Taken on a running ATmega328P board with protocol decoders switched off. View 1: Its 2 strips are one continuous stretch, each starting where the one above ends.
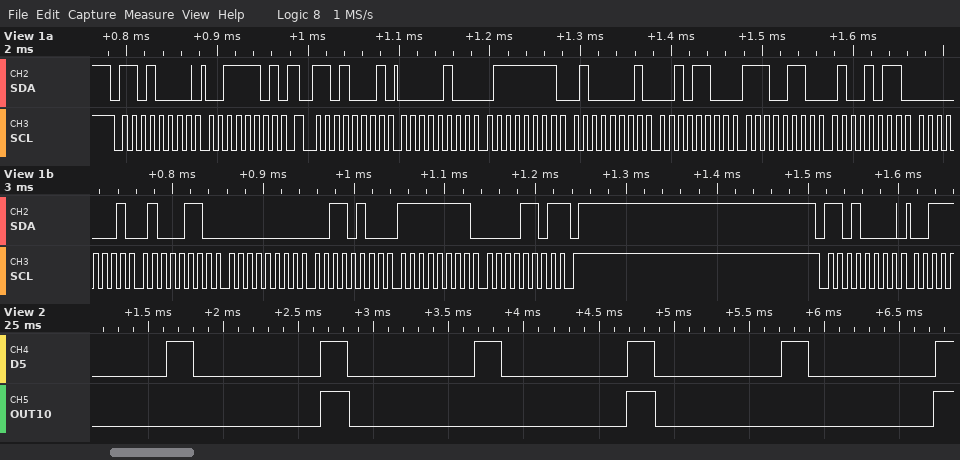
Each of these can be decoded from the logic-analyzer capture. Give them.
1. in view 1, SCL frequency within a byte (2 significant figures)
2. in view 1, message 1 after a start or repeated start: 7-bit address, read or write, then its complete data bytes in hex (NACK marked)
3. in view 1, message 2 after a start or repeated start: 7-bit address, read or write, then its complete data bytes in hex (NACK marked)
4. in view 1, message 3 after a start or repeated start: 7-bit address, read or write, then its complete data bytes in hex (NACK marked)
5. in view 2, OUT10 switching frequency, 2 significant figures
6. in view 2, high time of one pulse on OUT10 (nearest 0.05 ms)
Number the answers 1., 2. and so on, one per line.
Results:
1. 100 kHz
2. 0x68 write: 3D
3. 0x68 read: 04 7F 41 2C E6 4B 01 46 00 34 FF 0D NACK
4. 0x68 write
5. 490 Hz
6. 0.20 ms
